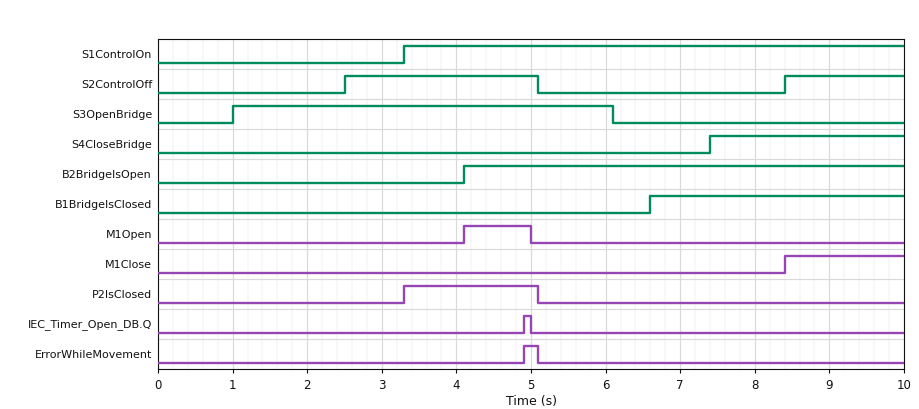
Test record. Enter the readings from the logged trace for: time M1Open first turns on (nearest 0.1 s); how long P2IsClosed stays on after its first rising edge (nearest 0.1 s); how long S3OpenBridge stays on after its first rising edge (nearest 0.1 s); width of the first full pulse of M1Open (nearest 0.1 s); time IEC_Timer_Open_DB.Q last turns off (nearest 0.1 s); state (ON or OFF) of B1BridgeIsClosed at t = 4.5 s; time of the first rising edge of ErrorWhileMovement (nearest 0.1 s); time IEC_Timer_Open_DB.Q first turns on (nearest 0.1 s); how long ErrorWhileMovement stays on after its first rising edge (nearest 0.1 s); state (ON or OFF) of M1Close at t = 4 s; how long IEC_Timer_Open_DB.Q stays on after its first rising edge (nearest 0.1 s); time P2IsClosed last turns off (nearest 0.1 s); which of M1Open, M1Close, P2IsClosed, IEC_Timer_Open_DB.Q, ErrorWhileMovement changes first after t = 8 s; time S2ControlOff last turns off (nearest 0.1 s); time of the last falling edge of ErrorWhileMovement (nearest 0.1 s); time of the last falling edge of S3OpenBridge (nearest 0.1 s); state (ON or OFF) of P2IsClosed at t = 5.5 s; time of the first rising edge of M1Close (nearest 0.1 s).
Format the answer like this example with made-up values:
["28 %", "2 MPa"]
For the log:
["4.1 s", "1.8 s", "5.1 s", "0.9 s", "5.0 s", "OFF", "4.9 s", "4.9 s", "0.2 s", "OFF", "0.1 s", "5.1 s", "M1Close", "5.1 s", "5.1 s", "6.1 s", "OFF", "8.4 s"]
